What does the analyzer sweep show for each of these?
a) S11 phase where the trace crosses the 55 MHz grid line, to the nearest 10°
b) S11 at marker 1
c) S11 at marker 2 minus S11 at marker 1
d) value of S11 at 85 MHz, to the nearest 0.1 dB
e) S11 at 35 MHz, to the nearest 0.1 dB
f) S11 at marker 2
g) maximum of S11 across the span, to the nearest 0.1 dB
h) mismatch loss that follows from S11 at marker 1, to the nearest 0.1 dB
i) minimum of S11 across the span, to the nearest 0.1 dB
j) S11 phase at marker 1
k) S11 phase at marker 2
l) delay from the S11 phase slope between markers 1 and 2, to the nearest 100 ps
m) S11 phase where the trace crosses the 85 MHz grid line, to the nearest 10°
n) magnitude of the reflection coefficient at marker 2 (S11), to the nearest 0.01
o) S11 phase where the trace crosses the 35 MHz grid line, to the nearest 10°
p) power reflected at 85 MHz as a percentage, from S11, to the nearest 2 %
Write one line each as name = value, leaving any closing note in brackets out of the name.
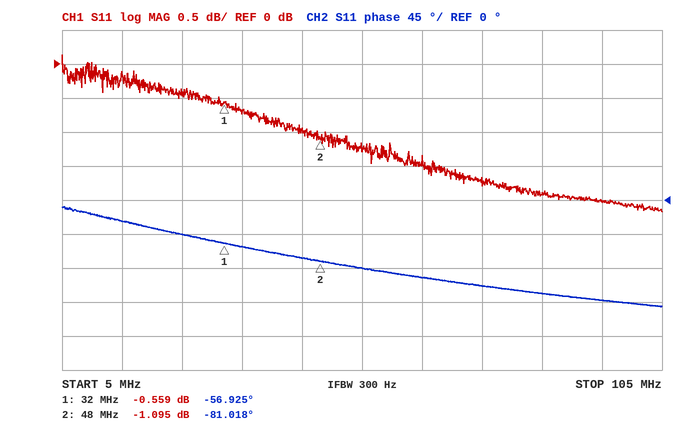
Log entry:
S11 phase where the trace crosses the 55 MHz grid line, to the nearest 10° = -90°
S11 at marker 1 = -0.559 dB
S11 at marker 2 minus S11 at marker 1 = -0.536 dB
value of S11 at 85 MHz, to the nearest 0.1 dB = -1.9 dB
S11 at 35 MHz, to the nearest 0.1 dB = -0.7 dB
S11 at marker 2 = -1.095 dB
maximum of S11 across the span, to the nearest 0.1 dB = 0.1 dB
mismatch loss that follows from S11 at marker 1, to the nearest 0.1 dB = 9.2 dB
minimum of S11 across the span, to the nearest 0.1 dB = -2.2 dB
S11 phase at marker 1 = -56.925°
S11 phase at marker 2 = -81.018°
delay from the S11 phase slope between markers 1 and 2, to the nearest 100 ps = 4.2 ns
S11 phase where the trace crosses the 85 MHz grid line, to the nearest 10° = -120°
magnitude of the reflection coefficient at marker 2 (S11), to the nearest 0.01 = 0.88
S11 phase where the trace crosses the 35 MHz grid line, to the nearest 10° = -60°
power reflected at 85 MHz as a percentage, from S11, to the nearest 2 % = 64 %
